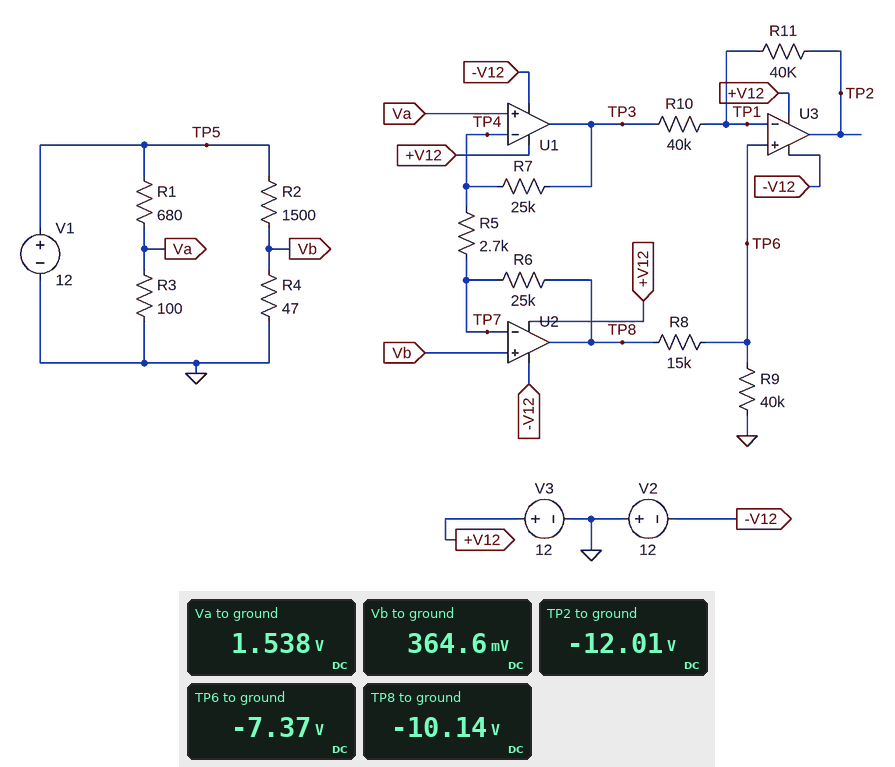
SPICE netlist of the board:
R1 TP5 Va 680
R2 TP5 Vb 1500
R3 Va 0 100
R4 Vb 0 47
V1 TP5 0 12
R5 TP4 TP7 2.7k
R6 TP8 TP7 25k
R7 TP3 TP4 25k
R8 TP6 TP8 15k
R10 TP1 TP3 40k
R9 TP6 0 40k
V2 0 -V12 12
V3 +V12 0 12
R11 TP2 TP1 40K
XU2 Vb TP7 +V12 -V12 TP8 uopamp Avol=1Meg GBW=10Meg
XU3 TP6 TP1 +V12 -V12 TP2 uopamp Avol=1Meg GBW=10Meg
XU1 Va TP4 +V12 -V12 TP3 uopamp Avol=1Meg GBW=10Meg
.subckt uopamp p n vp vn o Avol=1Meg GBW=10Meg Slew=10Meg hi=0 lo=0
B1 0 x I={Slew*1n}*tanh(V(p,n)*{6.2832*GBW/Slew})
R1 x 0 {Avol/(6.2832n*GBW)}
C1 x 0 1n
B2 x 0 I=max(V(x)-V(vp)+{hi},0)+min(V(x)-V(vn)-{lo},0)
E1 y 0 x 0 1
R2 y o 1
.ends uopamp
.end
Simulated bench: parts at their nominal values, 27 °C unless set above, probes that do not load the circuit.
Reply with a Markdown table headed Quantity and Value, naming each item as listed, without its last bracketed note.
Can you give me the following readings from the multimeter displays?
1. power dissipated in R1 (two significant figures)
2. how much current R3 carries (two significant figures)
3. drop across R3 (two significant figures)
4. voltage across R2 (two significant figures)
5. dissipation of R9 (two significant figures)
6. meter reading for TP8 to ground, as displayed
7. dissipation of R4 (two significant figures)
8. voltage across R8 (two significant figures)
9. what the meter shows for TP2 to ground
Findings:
| Quantity | Value |
|---|---|
| power dissipated in R1 | 160 mW |
| how much current R3 carries | 15 mA |
| drop across R3 | 1.5 V |
| voltage across R2 | 12 V |
| dissipation of R9 | 1.4 mW |
| meter reading for TP8 to ground, as displayed | -10.14 V |
| dissipation of R4 | 2.8 mW |
| voltage across R8 | 2.8 V |
| what the meter shows for TP2 to ground | -12.01 V |
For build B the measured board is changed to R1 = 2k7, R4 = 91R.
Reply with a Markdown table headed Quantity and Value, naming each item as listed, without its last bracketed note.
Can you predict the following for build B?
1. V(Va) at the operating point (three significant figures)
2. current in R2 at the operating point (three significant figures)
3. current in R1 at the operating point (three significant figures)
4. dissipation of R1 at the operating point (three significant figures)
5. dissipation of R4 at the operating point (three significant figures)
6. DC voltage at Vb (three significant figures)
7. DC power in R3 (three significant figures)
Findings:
| Quantity | Value |
|---|---|
| V(Va) at the operating point | 429 mV |
| current in R2 at the operating point | 7.54 mA |
| current in R1 at the operating point | 4.29 mA |
| dissipation of R1 at the operating point | 49.6 mW |
| dissipation of R4 at the operating point | 5.18 mW |
| DC voltage at Vb | 686 mV |
| DC power in R3 | 1.84 mW |
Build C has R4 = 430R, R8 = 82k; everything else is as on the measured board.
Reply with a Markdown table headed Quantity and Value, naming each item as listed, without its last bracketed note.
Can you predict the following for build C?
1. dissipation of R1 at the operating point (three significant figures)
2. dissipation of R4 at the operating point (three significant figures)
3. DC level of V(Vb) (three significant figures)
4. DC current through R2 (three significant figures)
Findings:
| Quantity | Value |
|---|---|
| dissipation of R1 at the operating point | 161 mW |
| dissipation of R4 at the operating point | 16.6 mW |
| DC level of V(Vb) | 2.67 V |
| DC current through R2 | 6.22 mA |
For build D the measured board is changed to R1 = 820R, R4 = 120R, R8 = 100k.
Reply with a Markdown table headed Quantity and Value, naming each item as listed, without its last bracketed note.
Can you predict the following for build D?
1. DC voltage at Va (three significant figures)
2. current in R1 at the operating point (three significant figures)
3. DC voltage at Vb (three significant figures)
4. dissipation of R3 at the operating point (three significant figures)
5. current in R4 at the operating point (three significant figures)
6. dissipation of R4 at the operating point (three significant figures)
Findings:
| Quantity | Value |
|---|---|
| DC voltage at Va | 1.30 V |
| current in R1 at the operating point | 13.0 mA |
| DC voltage at Vb | 889 mV |
| dissipation of R3 at the operating point | 17.0 mW |
| current in R4 at the operating point | 7.41 mA |
| dissipation of R4 at the operating point | 6.58 mW |
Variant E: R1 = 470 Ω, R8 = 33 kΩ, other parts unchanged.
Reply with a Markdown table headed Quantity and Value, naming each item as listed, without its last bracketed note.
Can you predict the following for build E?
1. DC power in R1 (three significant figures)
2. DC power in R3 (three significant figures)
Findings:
| Quantity | Value |
|---|---|
| DC power in R1 | 208 mW |
| DC power in R3 | 44.3 mW |
